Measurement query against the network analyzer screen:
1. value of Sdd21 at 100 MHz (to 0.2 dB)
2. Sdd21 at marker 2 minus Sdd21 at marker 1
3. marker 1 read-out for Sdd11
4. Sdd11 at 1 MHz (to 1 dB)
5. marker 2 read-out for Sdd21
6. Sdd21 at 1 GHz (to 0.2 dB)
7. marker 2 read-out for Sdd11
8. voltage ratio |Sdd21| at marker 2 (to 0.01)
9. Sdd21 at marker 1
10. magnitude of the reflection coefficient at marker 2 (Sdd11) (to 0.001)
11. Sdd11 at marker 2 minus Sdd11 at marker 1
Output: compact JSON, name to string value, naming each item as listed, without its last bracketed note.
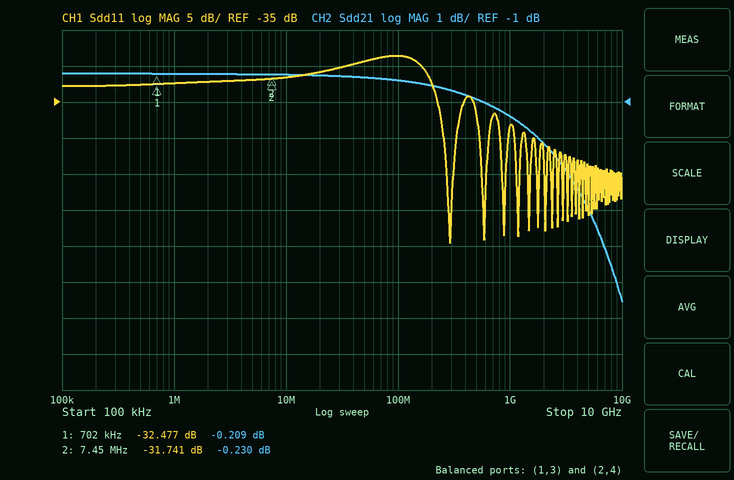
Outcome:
{"value of Sdd21 at 100 MHz": "-0.4 dB", "Sdd21 at marker 2 minus Sdd21 at marker 1": "-0.021 dB", "marker 1 read-out for Sdd11": "-32.477 dB", "Sdd11 at 1 MHz": "-32 dB", "marker 2 read-out for Sdd21": "-0.230 dB", "Sdd21 at 1 GHz": "-1.4 dB", "marker 2 read-out for Sdd11": "-31.741 dB", "voltage ratio |Sdd21| at marker 2": "0.97", "Sdd21 at marker 1": "-0.209 dB", "magnitude of the reflection coefficient at marker 2 (Sdd11)": "0.026", "Sdd11 at marker 2 minus Sdd11 at marker 1": "0.736 dB"}
